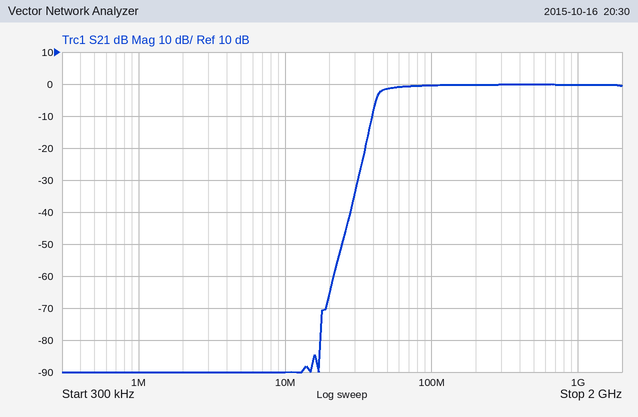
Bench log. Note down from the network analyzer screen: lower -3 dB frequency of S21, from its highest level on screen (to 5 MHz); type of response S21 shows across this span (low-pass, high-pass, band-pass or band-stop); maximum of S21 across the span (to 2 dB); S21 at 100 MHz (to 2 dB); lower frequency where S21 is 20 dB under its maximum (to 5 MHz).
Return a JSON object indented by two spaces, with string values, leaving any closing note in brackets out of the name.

{
  "lower -3 dB frequency of S21, from its highest level on screen": "45 MHz",
  "type of response S21 shows across this span": "high-pass",
  "maximum of S21 across the span": "0 dB",
  "S21 at 100 MHz": "0 dB",
  "lower frequency where S21 is 20 dB under its maximum": "35 MHz"
}
